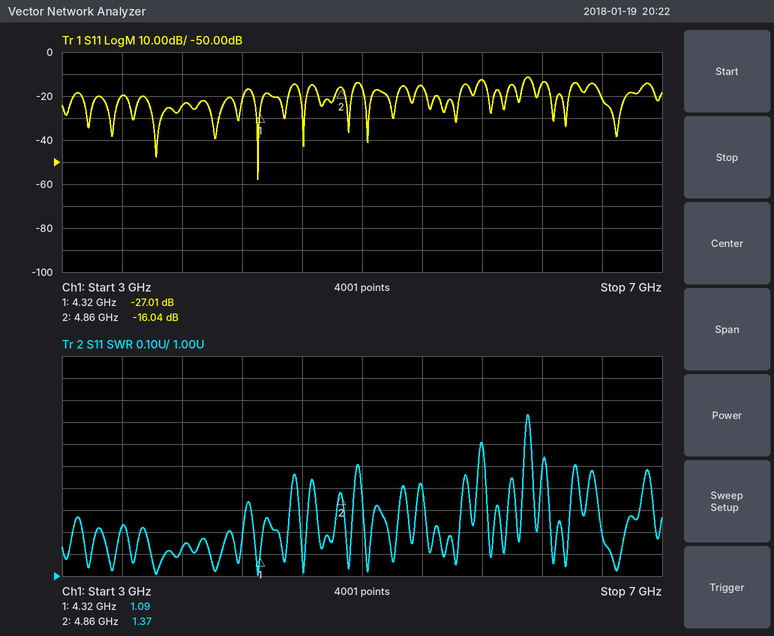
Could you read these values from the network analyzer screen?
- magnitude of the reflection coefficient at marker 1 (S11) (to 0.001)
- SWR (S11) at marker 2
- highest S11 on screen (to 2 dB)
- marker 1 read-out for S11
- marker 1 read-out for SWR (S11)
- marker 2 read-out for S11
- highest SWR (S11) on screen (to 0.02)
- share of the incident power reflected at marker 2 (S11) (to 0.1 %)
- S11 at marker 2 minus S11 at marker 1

0.045
1.37
-12 dB
-27.01 dB
1.09
-16.04 dB
1.74
2.5 %
10.97 dB
